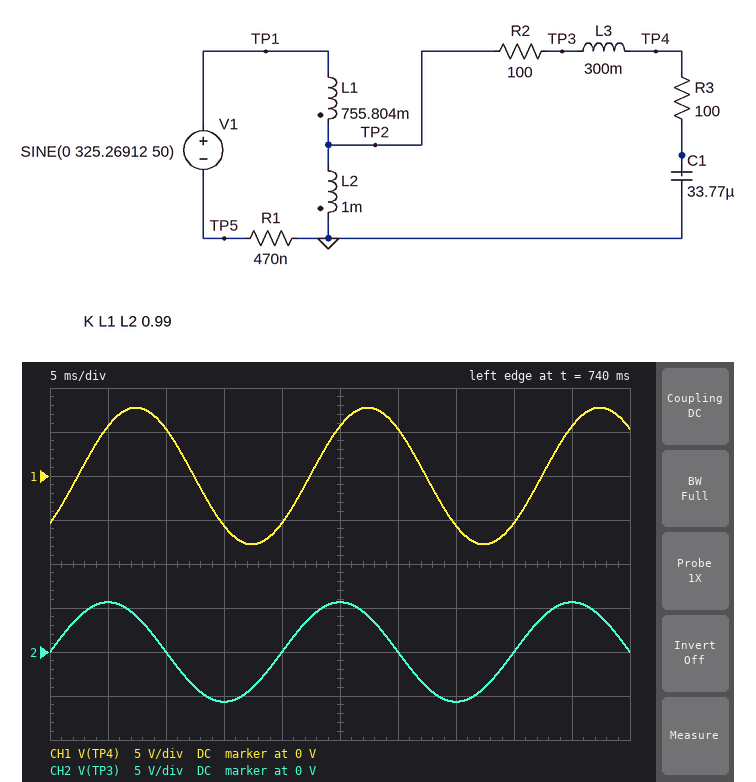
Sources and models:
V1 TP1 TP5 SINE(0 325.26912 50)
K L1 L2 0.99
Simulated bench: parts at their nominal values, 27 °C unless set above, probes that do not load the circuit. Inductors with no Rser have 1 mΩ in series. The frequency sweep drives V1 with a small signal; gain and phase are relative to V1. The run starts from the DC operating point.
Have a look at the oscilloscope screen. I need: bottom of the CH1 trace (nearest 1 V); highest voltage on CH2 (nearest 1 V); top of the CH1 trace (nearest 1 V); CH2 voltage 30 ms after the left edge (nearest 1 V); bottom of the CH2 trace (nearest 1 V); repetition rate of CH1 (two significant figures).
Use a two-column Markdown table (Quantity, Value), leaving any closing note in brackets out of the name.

| Quantity | Value |
|---|---|
| bottom of the CH1 trace | -8 V |
| highest voltage on CH2 | 6 V |
| top of the CH1 trace | 8 V |
| CH2 voltage 30 ms after the left edge | 0 V |
| bottom of the CH2 trace | -6 V |
| repetition rate of CH1 | 50 Hz |
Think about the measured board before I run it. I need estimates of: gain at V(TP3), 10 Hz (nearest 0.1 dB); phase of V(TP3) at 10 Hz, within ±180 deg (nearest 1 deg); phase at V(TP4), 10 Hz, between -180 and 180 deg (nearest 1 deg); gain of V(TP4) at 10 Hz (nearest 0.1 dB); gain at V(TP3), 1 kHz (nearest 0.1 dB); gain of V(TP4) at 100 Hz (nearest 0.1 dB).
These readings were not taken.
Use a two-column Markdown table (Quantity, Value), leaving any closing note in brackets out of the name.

| Quantity | Value |
|---|---|
| gain at V(TP3), 10 Hz | -29.7 dB |
| phase of V(TP3) at 10 Hz, within ±180 deg | -11 deg |
| phase at V(TP4), 10 Hz, between -180 and 180 deg | -12 deg |
| gain of V(TP4) at 10 Hz | -29.4 dB |
| gain at V(TP3), 1 kHz | -29.2 dB |
| gain of V(TP4) at 100 Hz | -36.1 dB |
